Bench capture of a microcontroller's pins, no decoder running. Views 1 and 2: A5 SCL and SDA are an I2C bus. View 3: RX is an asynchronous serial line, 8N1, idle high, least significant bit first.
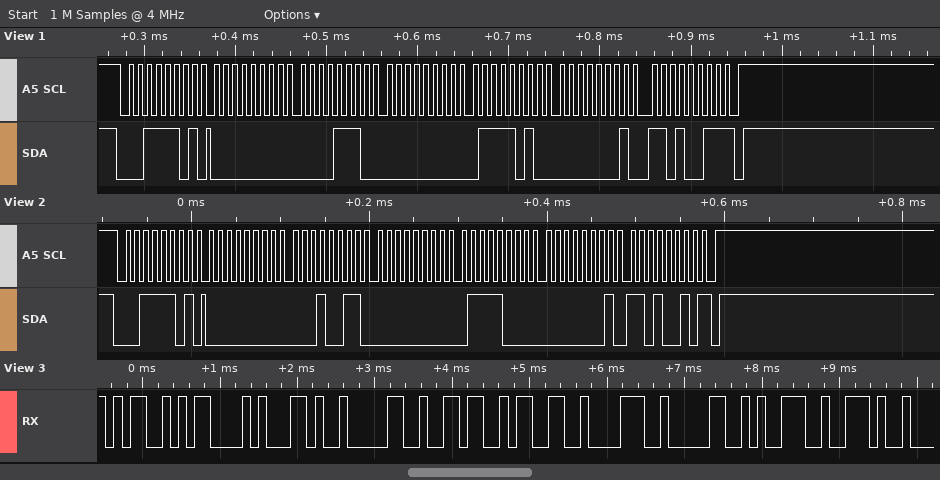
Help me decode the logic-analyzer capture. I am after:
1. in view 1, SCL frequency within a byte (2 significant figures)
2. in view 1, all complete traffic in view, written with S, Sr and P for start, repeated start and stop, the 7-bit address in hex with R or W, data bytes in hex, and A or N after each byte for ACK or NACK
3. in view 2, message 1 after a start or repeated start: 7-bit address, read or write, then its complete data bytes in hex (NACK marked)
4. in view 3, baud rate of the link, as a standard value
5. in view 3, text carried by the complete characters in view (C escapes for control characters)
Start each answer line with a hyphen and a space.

- 100 kHz
- S 1ER A 00 A 0E A 00 A 7A A 01 A D3 N P
- 0x1E read: 00 13 00 78 01 D2 NACK
- 9600 baud
- "MC,063809."
